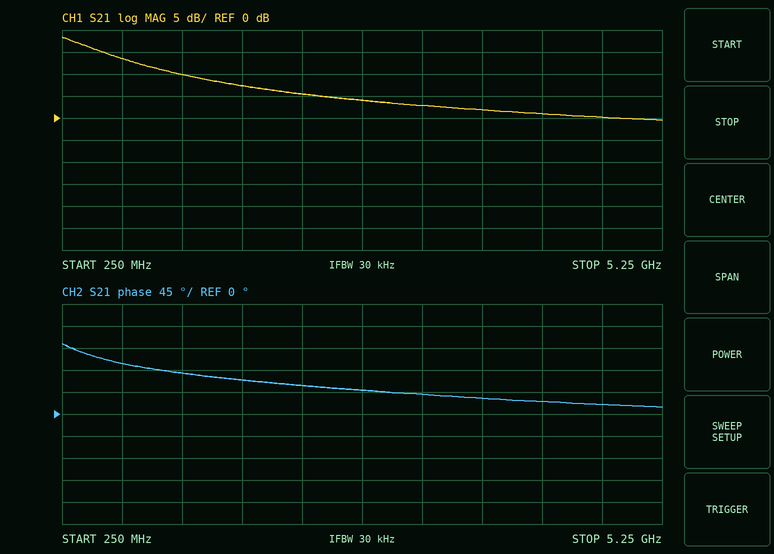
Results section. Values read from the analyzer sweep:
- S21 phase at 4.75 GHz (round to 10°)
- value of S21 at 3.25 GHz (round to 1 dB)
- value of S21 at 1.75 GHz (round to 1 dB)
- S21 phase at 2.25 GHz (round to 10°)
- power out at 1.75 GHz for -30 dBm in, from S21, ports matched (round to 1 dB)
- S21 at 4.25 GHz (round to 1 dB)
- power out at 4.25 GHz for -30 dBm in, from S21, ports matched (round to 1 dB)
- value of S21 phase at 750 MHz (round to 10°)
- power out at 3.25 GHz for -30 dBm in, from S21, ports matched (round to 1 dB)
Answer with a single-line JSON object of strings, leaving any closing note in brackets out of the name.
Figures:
{"S21 phase at 4.75 GHz": "20°", "value of S21 at 3.25 GHz": "3 dB", "value of S21 at 1.75 GHz": "7 dB", "S21 phase at 2.25 GHz": "60°", "power out at 1.75 GHz for -30 dBm in, from S21, ports matched": "-23 dBm", "S21 at 4.25 GHz": "1 dB", "power out at 4.25 GHz for -30 dBm in, from S21, ports matched": "-29 dBm", "value of S21 phase at 750 MHz": "100°", "power out at 3.25 GHz for -30 dBm in, from S21, ports matched": "-27 dBm"}
